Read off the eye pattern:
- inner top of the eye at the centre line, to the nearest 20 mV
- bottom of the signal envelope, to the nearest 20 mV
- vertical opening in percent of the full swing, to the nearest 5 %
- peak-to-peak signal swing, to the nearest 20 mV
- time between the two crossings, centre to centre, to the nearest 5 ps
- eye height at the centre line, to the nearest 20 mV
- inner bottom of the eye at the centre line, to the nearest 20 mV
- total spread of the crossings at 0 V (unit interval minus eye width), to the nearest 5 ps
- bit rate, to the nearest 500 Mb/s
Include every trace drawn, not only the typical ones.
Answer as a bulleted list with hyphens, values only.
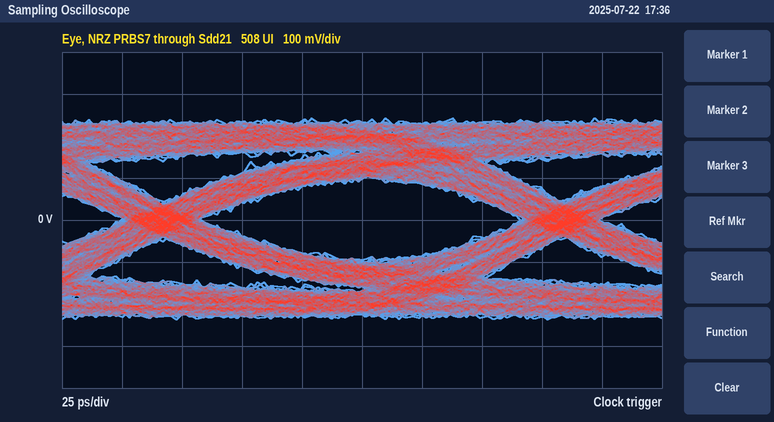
- 100 mV
- -240 mV
- 40 %
- 480 mV
- 165 ps
- 200 mV
- -100 mV
- 35 ps
- 6.0 Gb/s
